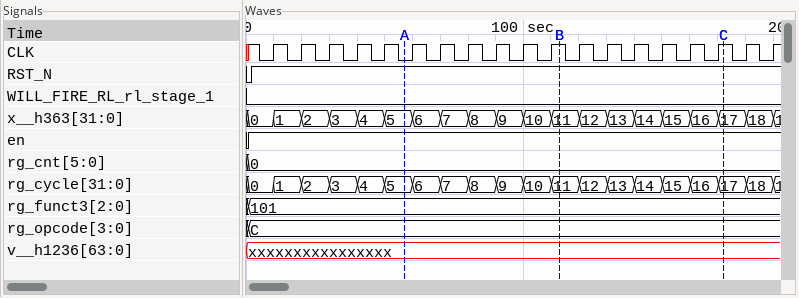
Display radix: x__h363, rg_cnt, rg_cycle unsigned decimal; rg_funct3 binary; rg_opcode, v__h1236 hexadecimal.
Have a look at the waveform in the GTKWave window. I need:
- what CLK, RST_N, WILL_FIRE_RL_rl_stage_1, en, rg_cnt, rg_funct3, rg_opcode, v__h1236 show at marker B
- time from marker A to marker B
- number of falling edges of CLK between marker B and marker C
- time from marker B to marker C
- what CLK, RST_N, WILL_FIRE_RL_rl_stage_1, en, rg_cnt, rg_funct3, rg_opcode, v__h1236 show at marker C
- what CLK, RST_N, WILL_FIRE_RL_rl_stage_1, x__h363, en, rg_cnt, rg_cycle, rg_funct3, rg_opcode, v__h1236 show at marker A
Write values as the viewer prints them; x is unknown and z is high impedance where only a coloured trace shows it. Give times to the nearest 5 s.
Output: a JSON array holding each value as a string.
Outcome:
["CLK=1, RST_N=1, WILL_FIRE_RL_rl_stage_1=0, en=1, rg_cnt=0, rg_funct3=101, rg_opcode=C, v__h1236=xxxxxxxxxxxxxxxx", "55 s", "6", "60 s", "CLK=1, RST_N=1, WILL_FIRE_RL_rl_stage_1=0, en=1, rg_cnt=0, rg_funct3=101, rg_opcode=C, v__h1236=xxxxxxxxxxxxxxxx", "CLK=0, RST_N=1, WILL_FIRE_RL_rl_stage_1=0, x__h363=5, en=1, rg_cnt=0, rg_cycle=5, rg_funct3=101, rg_opcode=C, v__h1236=xxxxxxxxxxxxxxxx"]
